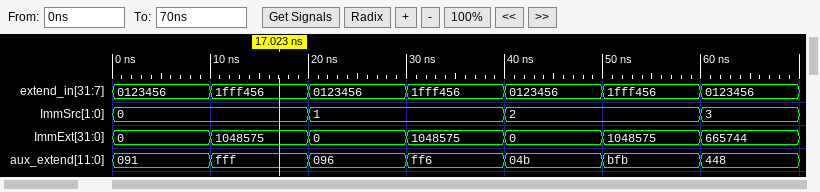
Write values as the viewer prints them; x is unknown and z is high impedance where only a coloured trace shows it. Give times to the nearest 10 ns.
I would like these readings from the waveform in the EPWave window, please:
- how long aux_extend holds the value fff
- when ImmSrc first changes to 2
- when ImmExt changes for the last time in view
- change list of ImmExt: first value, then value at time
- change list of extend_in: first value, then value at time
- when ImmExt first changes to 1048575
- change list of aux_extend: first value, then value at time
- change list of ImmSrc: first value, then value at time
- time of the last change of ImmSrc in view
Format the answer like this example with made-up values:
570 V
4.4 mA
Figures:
10 ns
40 ns
60 ns
0, 1048575 at 10 ns, 0 at 20 ns, 1048575 at 30 ns, 0 at 40 ns, 1048575 at 50 ns, 665744 at 60 ns
0123456, 1fff456 at 10 ns, 0123456 at 20 ns, 1fff456 at 30 ns, 0123456 at 40 ns, 1fff456 at 50 ns, 0123456 at 60 ns
10 ns
091, fff at 10 ns, 096 at 20 ns, ff6 at 30 ns, 04b at 40 ns, bfb at 50 ns, 448 at 60 ns
0, 1 at 20 ns, 2 at 40 ns, 3 at 60 ns
60 ns
